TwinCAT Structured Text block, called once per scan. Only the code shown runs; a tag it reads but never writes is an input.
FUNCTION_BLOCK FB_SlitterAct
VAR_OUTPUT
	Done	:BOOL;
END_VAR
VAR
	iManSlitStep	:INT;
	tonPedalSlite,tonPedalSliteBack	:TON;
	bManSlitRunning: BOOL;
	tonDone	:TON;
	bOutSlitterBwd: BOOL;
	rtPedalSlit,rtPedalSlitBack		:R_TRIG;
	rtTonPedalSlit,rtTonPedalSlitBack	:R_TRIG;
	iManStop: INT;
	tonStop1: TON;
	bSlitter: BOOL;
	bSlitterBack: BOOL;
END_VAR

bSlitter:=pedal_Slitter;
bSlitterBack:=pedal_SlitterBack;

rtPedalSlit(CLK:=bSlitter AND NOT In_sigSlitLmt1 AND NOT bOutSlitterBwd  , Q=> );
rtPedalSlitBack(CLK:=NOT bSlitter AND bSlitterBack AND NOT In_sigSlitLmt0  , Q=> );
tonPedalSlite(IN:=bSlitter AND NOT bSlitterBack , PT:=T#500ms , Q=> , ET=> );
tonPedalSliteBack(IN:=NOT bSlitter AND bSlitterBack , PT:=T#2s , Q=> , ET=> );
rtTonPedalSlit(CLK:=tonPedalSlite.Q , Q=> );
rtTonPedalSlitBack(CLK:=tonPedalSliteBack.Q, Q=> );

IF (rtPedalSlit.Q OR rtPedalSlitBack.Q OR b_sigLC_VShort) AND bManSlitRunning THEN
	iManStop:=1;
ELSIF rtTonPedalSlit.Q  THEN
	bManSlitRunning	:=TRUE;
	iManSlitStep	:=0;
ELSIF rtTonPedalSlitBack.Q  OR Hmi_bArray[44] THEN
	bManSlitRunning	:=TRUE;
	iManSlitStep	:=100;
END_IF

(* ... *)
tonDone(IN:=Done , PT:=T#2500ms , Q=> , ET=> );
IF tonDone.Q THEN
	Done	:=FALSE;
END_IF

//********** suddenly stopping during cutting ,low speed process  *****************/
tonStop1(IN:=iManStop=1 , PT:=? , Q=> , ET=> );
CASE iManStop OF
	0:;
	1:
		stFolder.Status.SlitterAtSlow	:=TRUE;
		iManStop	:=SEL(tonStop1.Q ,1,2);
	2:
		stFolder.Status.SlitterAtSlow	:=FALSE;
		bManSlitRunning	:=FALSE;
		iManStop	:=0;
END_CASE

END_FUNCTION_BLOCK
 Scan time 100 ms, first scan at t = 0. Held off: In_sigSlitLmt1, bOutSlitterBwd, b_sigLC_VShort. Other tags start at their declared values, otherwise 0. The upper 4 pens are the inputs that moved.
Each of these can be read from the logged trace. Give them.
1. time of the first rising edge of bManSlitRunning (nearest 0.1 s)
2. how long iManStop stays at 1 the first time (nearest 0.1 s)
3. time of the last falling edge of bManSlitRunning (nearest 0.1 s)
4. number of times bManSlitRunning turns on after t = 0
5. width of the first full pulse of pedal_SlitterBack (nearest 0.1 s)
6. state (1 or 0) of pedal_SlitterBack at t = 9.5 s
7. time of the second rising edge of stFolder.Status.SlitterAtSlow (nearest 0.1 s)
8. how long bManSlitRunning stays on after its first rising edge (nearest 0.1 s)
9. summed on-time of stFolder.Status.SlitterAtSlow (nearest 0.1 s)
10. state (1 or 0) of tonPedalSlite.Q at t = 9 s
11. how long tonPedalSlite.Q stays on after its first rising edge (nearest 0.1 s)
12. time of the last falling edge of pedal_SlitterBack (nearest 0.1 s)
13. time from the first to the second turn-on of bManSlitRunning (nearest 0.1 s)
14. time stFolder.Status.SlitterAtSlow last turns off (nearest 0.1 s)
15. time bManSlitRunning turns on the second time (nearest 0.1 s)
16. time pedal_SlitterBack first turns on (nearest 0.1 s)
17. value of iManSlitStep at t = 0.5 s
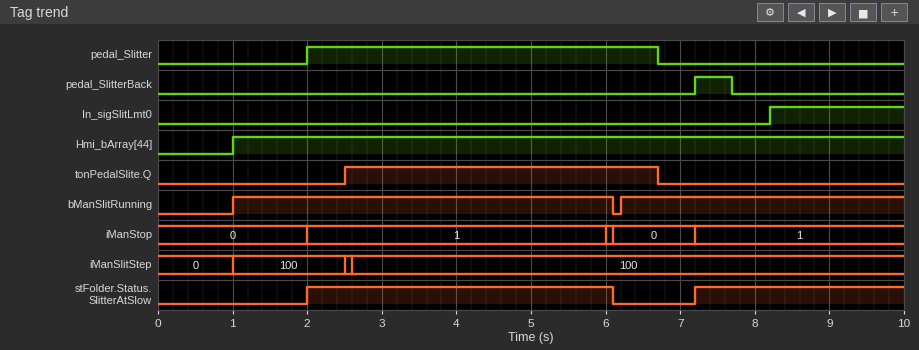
1.0 s
4.0 s
6.1 s
2
0.5 s
0
7.2 s
5.1 s
6.9 s
0
4.2 s
7.7 s
5.2 s
6.1 s
6.2 s
7.2 s
0
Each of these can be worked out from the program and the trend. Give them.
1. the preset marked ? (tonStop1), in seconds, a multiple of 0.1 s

4.0 s
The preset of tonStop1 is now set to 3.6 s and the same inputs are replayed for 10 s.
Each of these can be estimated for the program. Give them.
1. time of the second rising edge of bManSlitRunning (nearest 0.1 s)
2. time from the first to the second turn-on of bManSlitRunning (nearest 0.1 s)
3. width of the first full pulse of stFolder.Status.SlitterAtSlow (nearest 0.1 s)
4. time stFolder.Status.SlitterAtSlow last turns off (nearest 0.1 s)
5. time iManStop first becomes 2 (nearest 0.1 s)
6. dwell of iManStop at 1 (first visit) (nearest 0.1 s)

5.8 s
4.8 s
3.7 s
5.7 s
5.6 s
3.6 s
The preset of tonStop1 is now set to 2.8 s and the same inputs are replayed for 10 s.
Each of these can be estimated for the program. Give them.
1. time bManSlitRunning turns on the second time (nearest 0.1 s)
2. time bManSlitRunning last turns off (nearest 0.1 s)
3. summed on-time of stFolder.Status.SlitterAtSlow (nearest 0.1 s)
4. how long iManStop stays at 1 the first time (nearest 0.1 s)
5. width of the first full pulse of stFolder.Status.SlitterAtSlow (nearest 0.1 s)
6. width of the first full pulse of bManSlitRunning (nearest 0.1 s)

5.0 s
4.9 s
5.7 s
2.8 s
2.9 s
3.9 s
